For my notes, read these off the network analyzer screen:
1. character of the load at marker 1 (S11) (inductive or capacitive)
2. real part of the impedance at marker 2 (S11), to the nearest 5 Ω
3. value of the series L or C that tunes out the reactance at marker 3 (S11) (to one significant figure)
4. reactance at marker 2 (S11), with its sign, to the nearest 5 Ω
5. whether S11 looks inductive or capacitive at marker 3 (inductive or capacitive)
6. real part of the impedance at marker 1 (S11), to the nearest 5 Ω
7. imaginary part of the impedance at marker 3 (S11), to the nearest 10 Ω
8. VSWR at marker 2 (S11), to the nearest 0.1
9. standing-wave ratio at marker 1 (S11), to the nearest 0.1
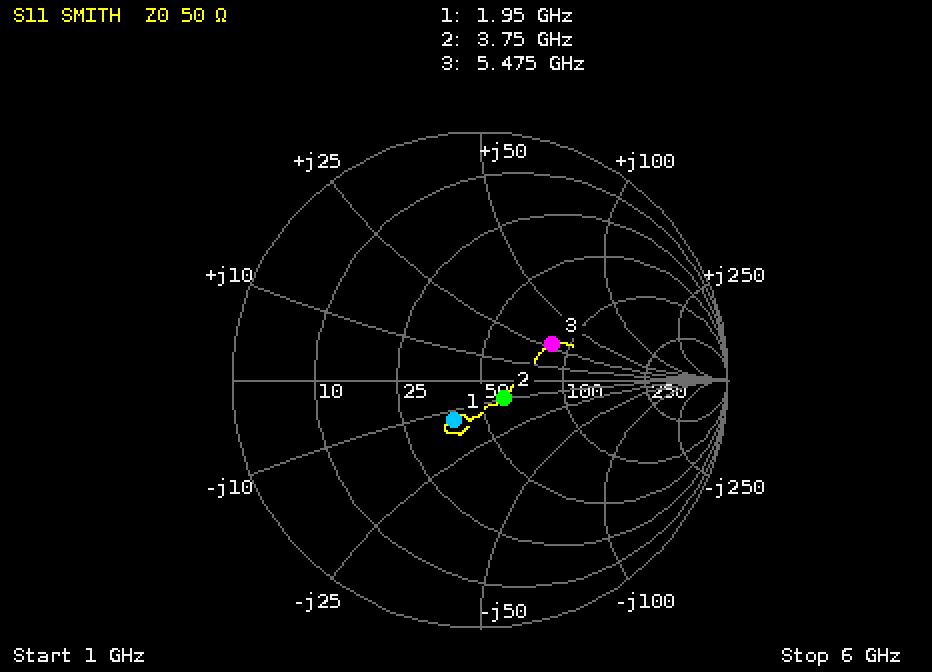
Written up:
capacitive
60 Ω
1 pF
-10 Ω
inductive
40 Ω
+30 Ω
1.3
1.5
